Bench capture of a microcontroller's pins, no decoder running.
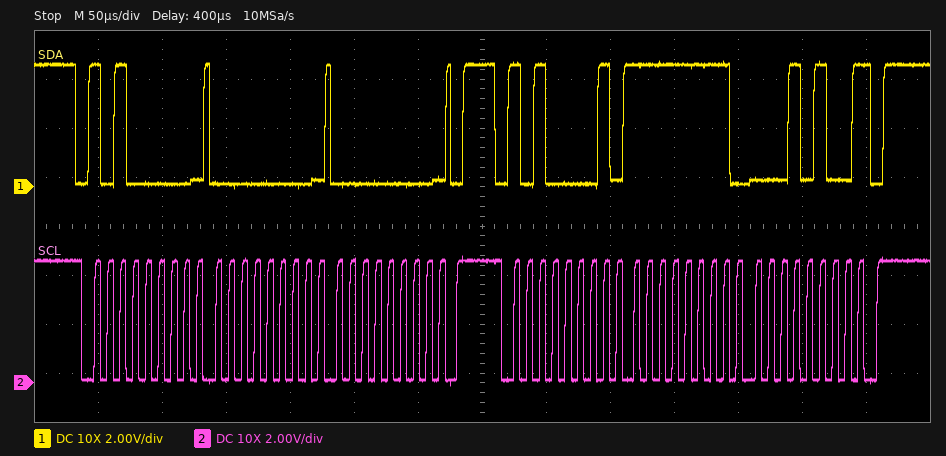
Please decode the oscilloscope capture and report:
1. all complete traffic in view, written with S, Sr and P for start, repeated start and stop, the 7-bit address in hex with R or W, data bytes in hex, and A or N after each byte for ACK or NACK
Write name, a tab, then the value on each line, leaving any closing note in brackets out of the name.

all complete traffic in view, written with S, Sr and P for start, repeated start and stop, the 7-bit address in hex with R or W, data bytes in hex, and A or N after each byte for ACK or NACK	S 50W A 00 A 00 A P S 50R A FF A 14 N P
